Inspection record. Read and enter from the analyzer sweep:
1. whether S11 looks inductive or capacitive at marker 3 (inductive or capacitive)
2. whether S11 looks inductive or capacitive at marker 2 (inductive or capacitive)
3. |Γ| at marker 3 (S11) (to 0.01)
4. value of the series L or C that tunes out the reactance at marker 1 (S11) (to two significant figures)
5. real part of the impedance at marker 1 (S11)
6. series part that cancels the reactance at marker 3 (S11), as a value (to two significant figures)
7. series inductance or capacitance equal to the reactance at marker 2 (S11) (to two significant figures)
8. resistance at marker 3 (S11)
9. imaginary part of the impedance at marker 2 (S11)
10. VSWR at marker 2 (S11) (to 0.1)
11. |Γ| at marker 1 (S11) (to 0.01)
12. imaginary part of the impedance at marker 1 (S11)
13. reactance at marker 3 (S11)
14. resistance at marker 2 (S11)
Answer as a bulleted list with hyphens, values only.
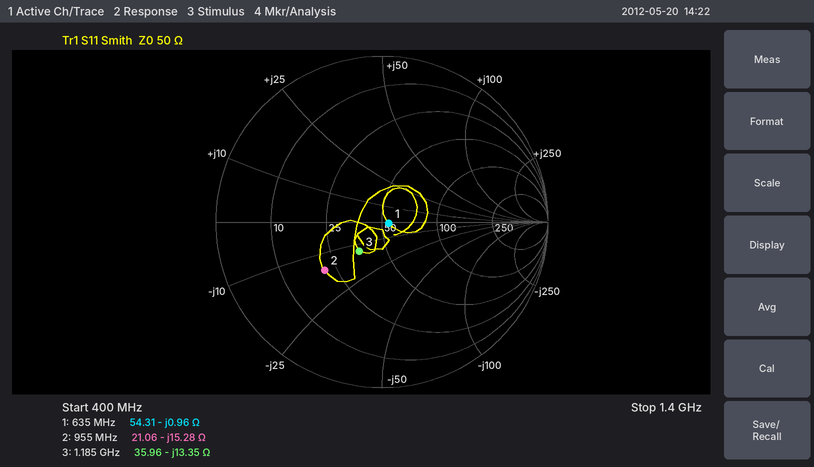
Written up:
- capacitive
- capacitive
- 0.22
- 240 pH
- 54.31 Ω
- 1.8 nH
- 11 pF
- 35.96 Ω
- -15.28 Ω
- 2.6
- 0.04
- -0.96 Ω
- -13.35 Ω
- 21.06 Ω
